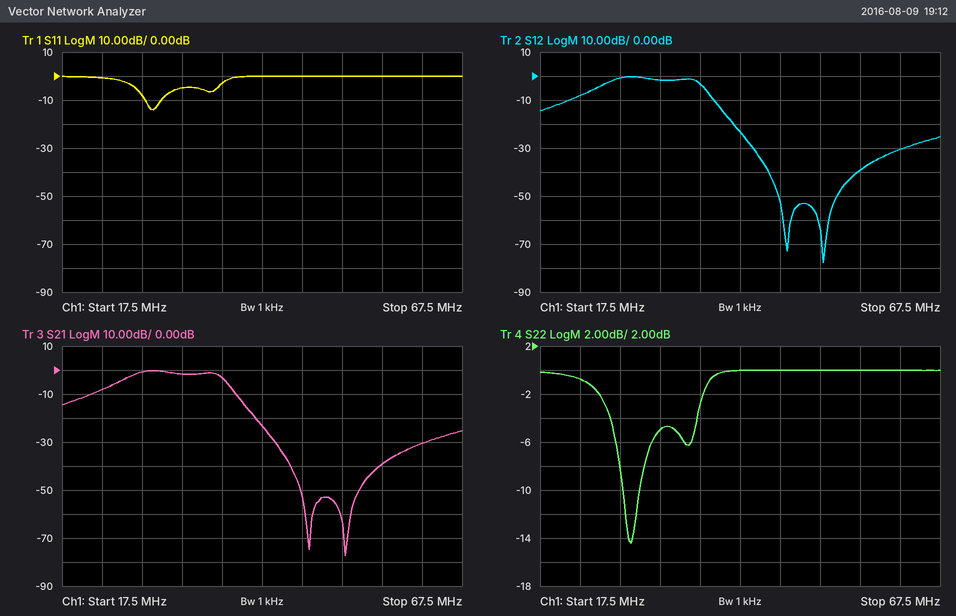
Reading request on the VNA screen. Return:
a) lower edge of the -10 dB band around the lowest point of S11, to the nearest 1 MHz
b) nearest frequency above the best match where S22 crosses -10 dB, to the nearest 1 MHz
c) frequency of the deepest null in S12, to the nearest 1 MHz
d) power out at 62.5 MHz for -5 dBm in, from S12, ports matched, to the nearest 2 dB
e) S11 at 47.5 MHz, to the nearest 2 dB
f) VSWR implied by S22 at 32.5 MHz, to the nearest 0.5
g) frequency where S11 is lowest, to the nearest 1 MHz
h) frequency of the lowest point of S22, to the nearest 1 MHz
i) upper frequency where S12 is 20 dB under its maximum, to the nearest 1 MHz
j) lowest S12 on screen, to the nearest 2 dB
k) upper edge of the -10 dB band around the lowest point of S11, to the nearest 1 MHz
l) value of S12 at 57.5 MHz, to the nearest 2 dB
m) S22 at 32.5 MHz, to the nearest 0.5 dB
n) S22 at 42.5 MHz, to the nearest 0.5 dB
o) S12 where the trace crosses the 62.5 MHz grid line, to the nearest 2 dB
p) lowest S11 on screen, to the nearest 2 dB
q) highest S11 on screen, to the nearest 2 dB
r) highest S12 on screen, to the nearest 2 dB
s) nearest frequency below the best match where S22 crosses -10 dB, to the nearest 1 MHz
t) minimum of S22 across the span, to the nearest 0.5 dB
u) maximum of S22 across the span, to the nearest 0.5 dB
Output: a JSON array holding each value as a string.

["28 MHz", "30 MHz", "53 MHz", "-36 dBm", "0 dB", "3.5", "29 MHz", "29 MHz", "42 MHz", "-78 dB", "30 MHz", "-40 dB", "-5.0 dB", "0.0 dB", "-30 dB", "-14 dB", "0 dB", "0 dB", "28 MHz", "-14.5 dB", "0.0 dB"]
